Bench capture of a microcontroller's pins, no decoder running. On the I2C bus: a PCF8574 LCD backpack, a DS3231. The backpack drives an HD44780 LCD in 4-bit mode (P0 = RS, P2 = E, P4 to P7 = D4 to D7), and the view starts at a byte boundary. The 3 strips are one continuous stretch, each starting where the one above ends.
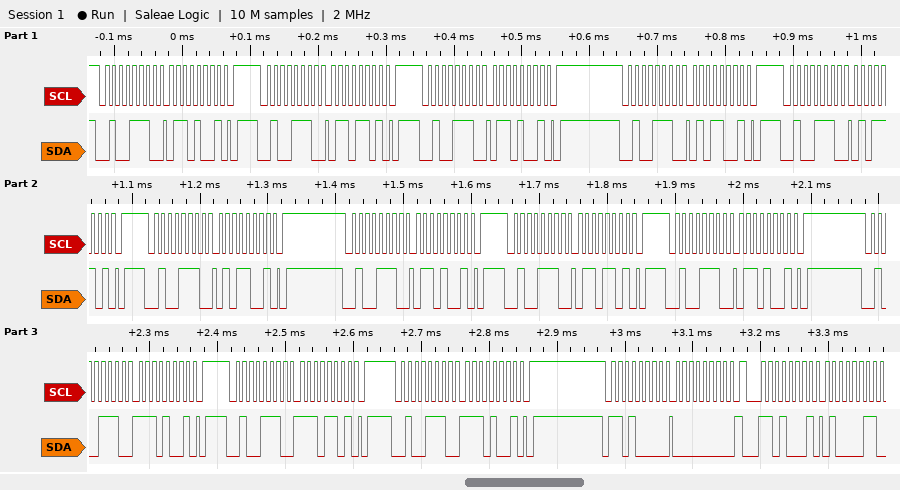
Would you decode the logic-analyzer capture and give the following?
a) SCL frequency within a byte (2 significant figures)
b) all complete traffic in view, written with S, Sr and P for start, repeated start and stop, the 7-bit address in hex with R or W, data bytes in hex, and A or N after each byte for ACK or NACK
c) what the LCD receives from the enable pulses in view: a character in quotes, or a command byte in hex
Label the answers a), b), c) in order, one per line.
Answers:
a) 100 kHz
b) S 27W A 69 A P S 27W A 6D A P S 27W A 69 A P S 27W A 59 A P S 27W A 5D A P S 27W A 59 A P S 27W A 69 A P S 27W A 6D A P S 27W A 69 A P S 27W A E9 A P S 27W A ED A P S 27W A E9 A P S 68W A 00 A Sr 68R A 43 A
c) 'e' 'n'
